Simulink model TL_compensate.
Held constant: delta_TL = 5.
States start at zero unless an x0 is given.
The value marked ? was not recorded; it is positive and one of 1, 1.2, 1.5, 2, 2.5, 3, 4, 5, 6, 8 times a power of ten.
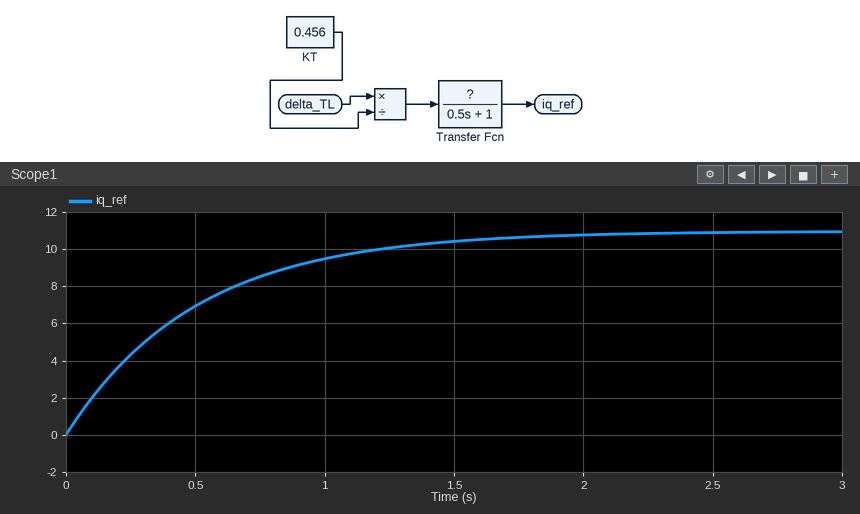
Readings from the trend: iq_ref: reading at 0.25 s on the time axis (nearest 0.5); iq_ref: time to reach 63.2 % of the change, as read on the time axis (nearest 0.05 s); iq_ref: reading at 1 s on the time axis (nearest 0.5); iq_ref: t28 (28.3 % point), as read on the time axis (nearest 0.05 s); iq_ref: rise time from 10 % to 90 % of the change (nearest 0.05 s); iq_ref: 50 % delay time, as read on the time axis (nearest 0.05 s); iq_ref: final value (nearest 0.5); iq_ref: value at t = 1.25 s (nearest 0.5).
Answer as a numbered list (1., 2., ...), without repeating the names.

1. 4.5
2. 0.50 s
3. 9.5
4. 0.15 s
5. 1.10 s
6. 0.35 s
7. 11.0
8. 10.0
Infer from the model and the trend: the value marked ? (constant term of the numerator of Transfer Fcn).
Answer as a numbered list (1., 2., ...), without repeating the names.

1. 1
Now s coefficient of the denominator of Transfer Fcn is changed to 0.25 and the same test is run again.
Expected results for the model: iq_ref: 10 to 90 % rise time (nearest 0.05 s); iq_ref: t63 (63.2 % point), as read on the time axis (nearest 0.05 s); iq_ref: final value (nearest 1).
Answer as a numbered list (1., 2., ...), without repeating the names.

1. 0.55 s
2. 0.25 s
3. 11
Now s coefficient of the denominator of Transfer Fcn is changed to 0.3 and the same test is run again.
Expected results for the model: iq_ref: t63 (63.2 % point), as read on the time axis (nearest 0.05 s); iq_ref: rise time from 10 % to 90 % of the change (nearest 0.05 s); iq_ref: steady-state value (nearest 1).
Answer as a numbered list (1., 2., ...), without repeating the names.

1. 0.30 s
2. 0.65 s
3. 11
